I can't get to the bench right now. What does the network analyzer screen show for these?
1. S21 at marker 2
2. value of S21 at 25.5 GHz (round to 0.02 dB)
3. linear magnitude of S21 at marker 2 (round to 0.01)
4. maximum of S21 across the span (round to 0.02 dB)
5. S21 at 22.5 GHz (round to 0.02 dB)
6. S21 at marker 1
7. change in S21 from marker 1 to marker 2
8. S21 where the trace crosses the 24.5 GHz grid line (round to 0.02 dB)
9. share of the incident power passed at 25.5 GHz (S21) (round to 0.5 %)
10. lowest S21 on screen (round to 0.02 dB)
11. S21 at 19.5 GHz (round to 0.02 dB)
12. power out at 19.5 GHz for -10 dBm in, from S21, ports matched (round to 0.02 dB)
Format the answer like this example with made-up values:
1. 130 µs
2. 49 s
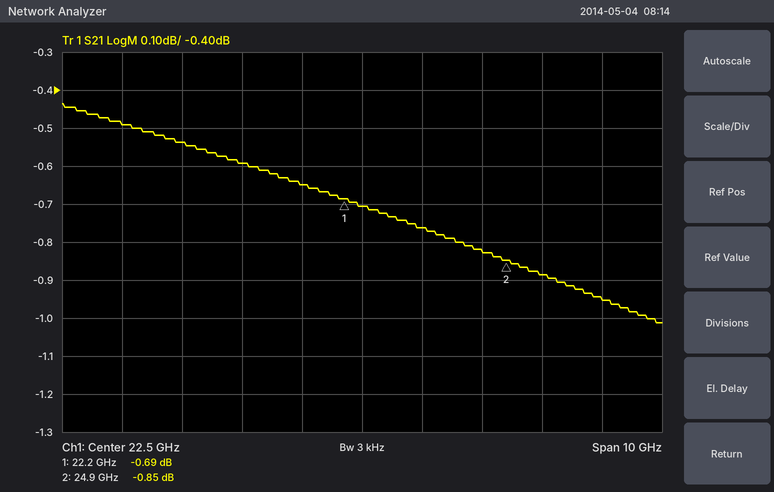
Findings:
1. -0.85 dB
2. -0.88 dB
3. 0.91
4. -0.44 dB
5. -0.70 dB
6. -0.69 dB
7. -0.16 dB
8. -0.82 dB
9. 81.5 %
10. -1.02 dB
11. -0.54 dB
12. -10.54 dBm
